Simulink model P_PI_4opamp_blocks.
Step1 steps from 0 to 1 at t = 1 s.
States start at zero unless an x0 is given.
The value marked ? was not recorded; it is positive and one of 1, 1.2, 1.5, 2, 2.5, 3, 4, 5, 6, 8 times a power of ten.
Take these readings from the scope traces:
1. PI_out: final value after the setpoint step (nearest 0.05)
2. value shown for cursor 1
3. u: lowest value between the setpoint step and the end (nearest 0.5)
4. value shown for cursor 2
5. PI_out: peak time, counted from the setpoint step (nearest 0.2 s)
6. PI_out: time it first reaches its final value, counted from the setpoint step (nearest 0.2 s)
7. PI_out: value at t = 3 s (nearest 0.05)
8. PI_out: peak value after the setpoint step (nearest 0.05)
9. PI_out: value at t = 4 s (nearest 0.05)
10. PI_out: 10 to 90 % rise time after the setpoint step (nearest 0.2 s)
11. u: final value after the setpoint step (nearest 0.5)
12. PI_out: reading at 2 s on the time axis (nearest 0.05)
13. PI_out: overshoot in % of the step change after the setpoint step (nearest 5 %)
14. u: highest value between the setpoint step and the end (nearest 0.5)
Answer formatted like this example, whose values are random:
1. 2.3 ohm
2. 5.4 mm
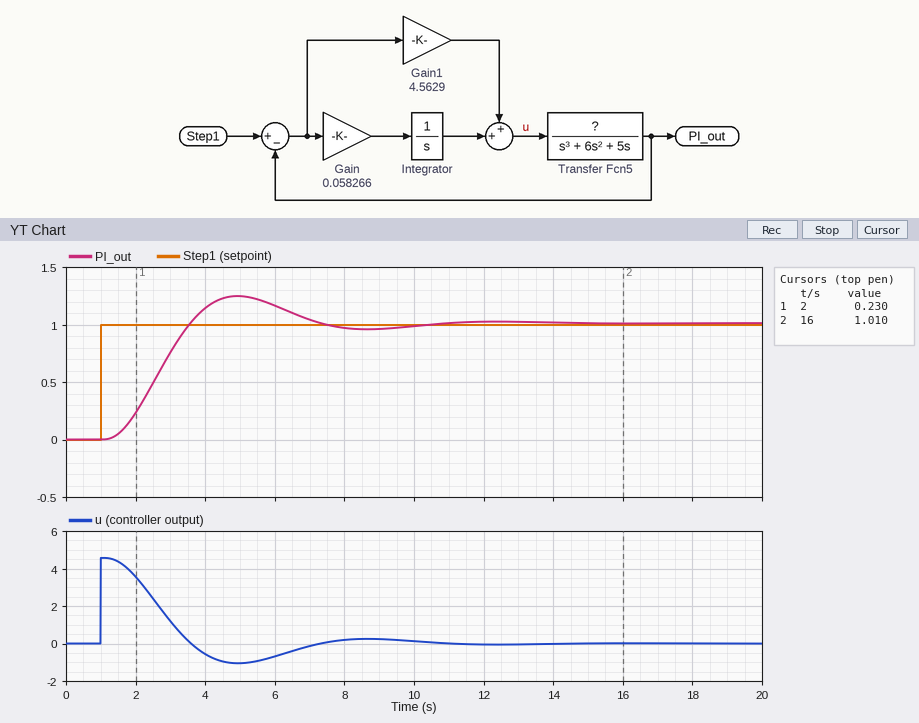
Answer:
1. 1.00
2. 0.230
3. -1.0
4. 1.010
5. 4.0 s
6. 2.6 s
7. 0.75
8. 1.25
9. 1.15
10. 1.6 s
11. 0.0
12. 0.25
13. 25 %
14. 4.5
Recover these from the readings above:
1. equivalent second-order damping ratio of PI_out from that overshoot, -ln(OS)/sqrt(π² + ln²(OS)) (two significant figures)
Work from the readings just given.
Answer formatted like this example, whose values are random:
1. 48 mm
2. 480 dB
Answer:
1. 0.40
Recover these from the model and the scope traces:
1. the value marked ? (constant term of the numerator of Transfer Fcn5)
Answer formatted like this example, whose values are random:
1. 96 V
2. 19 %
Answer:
1. 1
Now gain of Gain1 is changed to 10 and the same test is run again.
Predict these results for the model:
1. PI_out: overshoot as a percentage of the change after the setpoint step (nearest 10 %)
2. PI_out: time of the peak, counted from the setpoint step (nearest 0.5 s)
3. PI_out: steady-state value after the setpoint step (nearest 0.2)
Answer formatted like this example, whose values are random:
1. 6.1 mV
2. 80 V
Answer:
1. 50 %
2. 2.5 s
3. 1.0
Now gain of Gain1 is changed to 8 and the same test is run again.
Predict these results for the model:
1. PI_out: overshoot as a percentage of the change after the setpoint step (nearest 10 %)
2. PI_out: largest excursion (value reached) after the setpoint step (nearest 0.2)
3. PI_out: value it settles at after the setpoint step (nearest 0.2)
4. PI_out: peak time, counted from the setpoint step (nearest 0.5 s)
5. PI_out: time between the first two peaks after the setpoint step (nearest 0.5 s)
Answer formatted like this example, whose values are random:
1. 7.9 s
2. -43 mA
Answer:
1. 40 %
2. 1.4
3. 1.0
4. 3.0 s
5. 5.5 s
